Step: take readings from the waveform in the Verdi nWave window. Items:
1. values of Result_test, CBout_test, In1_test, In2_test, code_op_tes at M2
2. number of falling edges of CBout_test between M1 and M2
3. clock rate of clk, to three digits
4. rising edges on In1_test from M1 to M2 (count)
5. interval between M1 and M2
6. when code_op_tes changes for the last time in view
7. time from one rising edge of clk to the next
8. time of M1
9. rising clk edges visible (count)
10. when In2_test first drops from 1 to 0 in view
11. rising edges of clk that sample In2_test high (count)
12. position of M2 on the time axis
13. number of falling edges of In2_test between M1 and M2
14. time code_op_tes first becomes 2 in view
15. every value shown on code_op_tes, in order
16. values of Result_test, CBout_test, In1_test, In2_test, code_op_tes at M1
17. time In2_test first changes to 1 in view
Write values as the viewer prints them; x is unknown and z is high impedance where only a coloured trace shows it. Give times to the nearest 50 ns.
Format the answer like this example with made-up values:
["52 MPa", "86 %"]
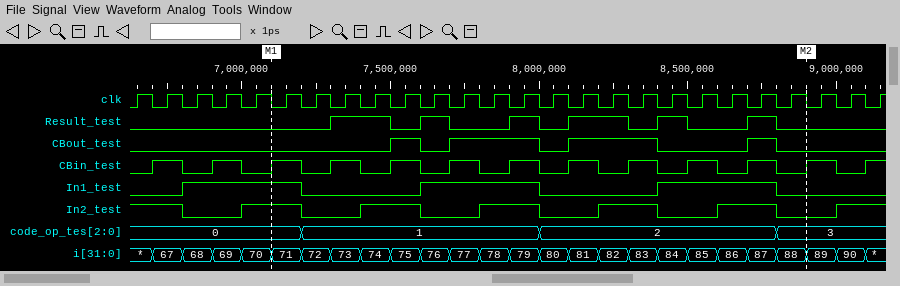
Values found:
["Result_test=0, CBout_test=0, In1_test=0, In2_test=0, code_op_tes=3", "4", "10.0 MHz", "2", "1800 ns", "8800 ns", "100 ns", "7100 ns", "26", "6800 ns", "14", "8900 ns", "5", "8000 ns", "0, 1, 2, 3", "Result_test=0, CBout_test=0, In1_test=1, In2_test=1, code_op_tes=0", "7000 ns"]
